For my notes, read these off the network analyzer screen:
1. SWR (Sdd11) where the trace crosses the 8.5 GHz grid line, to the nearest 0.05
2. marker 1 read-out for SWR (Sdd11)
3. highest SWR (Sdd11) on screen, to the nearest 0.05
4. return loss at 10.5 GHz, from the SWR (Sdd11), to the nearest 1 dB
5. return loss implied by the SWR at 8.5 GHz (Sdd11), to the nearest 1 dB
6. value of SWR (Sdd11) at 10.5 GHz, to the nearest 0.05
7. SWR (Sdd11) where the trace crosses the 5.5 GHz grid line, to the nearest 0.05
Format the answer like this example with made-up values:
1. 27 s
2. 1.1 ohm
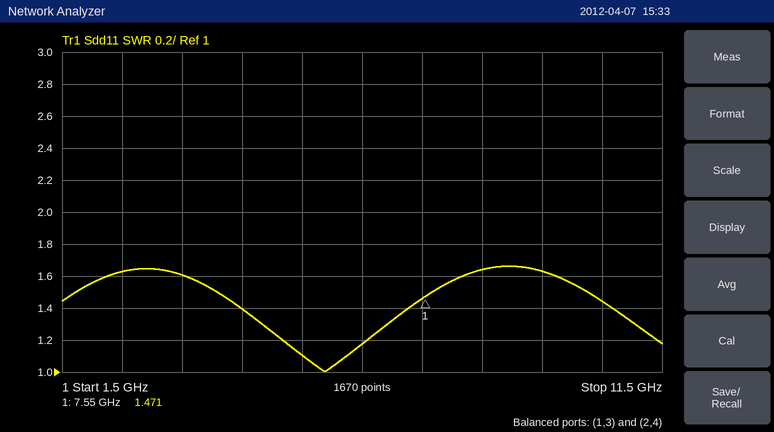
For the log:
1. 1.65
2. 1.471
3. 1.65
4. 15 dB
5. 12 dB
6. 1.45
7. 1.10
